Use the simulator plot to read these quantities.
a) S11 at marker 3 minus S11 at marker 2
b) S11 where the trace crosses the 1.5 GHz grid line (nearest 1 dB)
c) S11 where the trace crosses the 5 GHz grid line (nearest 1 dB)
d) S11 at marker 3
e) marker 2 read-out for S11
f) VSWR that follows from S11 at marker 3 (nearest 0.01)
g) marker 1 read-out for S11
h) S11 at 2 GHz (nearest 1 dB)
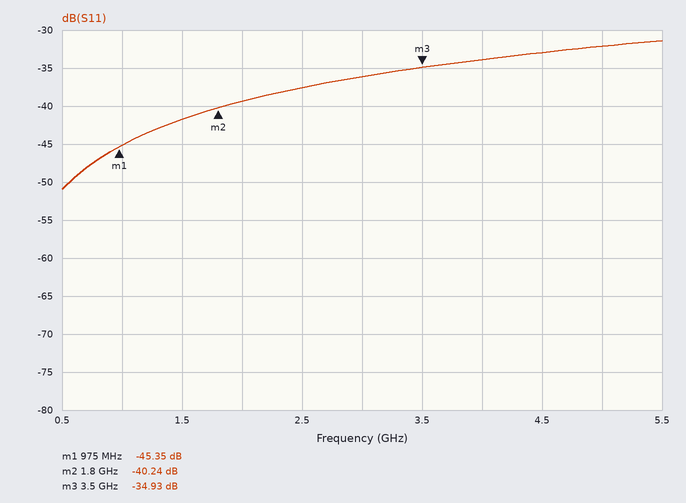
5.31 dB
-42 dB
-32 dB
-34.93 dB
-40.24 dB
1.04
-45.35 dB
-39 dB
